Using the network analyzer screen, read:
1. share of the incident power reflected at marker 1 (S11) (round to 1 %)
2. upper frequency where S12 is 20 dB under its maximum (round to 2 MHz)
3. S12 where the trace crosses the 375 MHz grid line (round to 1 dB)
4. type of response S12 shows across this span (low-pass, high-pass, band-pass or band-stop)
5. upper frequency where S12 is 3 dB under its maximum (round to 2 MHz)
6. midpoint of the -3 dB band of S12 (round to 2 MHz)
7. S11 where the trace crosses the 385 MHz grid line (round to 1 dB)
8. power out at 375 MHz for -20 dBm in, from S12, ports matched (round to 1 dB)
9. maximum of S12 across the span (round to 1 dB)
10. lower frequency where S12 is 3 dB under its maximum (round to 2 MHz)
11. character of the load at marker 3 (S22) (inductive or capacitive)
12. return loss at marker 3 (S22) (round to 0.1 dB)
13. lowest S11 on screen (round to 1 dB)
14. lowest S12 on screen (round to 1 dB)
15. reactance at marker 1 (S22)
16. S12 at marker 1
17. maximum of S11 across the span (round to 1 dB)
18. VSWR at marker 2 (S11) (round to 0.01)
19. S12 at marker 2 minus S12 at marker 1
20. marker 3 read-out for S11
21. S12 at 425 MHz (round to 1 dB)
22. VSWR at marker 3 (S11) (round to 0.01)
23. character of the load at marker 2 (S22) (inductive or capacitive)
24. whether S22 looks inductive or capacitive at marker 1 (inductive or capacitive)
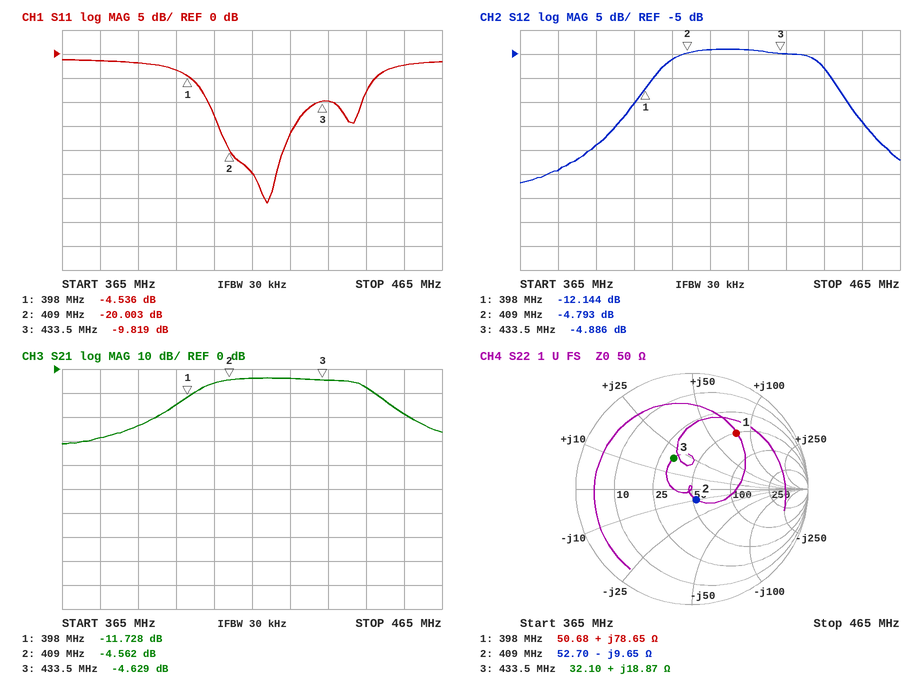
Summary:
35 %
460 MHz
-29 dB
band-pass
444 MHz
424 MHz
-2 dB
-49 dBm
-4 dB
404 MHz
inductive
10.2 dB
-31 dB
-32 dB
+78.65 Ω
-12.144 dB
-1 dB
1.22
7.351 dB
-9.819 dB
-4 dB
1.95
capacitive
inductive
